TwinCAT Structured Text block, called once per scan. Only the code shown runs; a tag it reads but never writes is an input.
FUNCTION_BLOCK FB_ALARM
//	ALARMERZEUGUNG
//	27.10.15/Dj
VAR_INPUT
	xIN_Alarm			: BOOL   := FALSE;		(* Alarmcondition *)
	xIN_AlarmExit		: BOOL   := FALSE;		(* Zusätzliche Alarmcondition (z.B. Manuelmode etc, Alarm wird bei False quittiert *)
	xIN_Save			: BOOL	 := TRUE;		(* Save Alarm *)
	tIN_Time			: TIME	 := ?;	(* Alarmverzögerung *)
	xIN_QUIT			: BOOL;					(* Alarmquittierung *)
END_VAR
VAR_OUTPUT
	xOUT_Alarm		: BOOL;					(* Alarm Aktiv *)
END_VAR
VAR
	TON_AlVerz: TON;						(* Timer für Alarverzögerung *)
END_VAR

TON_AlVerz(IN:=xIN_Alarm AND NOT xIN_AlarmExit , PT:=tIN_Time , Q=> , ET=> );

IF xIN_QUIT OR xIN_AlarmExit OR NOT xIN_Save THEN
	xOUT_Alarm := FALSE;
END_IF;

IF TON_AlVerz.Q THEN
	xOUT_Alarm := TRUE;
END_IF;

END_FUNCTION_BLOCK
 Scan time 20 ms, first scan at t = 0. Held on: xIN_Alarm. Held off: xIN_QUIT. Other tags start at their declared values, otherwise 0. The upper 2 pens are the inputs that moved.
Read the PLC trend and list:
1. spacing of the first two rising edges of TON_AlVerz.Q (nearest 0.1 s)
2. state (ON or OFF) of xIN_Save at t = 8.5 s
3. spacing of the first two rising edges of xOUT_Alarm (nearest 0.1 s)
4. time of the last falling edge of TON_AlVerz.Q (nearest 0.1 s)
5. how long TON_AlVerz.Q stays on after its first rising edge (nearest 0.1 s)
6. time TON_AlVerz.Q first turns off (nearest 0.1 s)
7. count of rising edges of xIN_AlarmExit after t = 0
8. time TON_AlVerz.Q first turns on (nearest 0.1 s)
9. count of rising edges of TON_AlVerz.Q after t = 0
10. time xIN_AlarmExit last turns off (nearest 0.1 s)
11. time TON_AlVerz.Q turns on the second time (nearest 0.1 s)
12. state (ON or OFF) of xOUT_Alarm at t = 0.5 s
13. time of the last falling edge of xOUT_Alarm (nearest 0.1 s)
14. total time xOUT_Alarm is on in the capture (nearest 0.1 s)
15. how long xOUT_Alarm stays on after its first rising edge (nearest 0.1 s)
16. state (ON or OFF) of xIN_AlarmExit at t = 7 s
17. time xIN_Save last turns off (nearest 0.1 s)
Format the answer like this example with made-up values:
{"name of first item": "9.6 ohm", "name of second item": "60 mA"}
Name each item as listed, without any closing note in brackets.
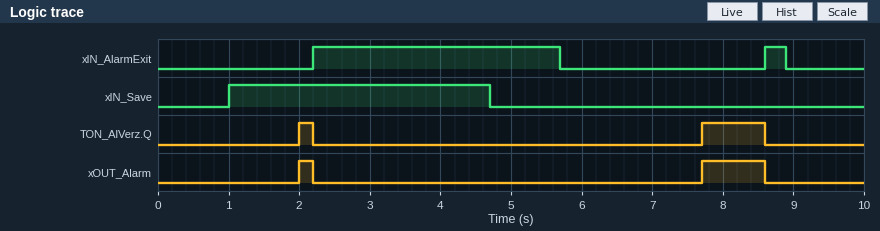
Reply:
{"spacing of the first two rising edges of TON_AlVerz.Q": "5.7 s", "state (ON or OFF) of xIN_Save at t = 8.5 s": "OFF", "spacing of the first two rising edges of xOUT_Alarm": "5.7 s", "time of the last falling edge of TON_AlVerz.Q": "8.6 s", "how long TON_AlVerz.Q stays on after its first rising edge": "0.2 s", "time TON_AlVerz.Q first turns off": "2.2 s", "count of rising edges of xIN_AlarmExit after t = 0": "2", "time TON_AlVerz.Q first turns on": "2.0 s", "count of rising edges of TON_AlVerz.Q after t = 0": "2", "time xIN_AlarmExit last turns off": "8.9 s", "time TON_AlVerz.Q turns on the second time": "7.7 s", "state (ON or OFF) of xOUT_Alarm at t = 0.5 s": "OFF", "time of the last falling edge of xOUT_Alarm": "8.6 s", "total time xOUT_Alarm is on in the capture": "1.1 s", "how long xOUT_Alarm stays on after its first rising edge": "0.2 s", "state (ON or OFF) of xIN_AlarmExit at t = 7 s": "OFF", "time xIN_Save last turns off": "4.7 s"}
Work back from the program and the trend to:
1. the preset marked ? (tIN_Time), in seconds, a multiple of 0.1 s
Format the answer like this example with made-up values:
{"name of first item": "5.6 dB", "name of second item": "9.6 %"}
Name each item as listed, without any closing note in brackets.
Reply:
{"the preset marked ? (tIN_Time), in seconds, a multiple of 0.1 s": "2.0 s"}
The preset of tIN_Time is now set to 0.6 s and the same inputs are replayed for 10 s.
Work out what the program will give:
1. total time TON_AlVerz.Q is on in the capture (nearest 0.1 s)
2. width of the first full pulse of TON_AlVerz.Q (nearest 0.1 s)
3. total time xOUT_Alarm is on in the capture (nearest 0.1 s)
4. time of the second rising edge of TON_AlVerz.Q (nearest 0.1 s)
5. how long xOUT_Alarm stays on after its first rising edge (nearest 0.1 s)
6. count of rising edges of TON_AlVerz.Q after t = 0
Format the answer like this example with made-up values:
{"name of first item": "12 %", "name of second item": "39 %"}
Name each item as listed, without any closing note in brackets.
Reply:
{"total time TON_AlVerz.Q is on in the capture": "4.4 s", "width of the first full pulse of TON_AlVerz.Q": "1.6 s", "total time xOUT_Alarm is on in the capture": "4.4 s", "time of the second rising edge of TON_AlVerz.Q": "6.3 s", "how long xOUT_Alarm stays on after its first rising edge": "1.6 s", "count of rising edges of TON_AlVerz.Q after t = 0": "3"}
